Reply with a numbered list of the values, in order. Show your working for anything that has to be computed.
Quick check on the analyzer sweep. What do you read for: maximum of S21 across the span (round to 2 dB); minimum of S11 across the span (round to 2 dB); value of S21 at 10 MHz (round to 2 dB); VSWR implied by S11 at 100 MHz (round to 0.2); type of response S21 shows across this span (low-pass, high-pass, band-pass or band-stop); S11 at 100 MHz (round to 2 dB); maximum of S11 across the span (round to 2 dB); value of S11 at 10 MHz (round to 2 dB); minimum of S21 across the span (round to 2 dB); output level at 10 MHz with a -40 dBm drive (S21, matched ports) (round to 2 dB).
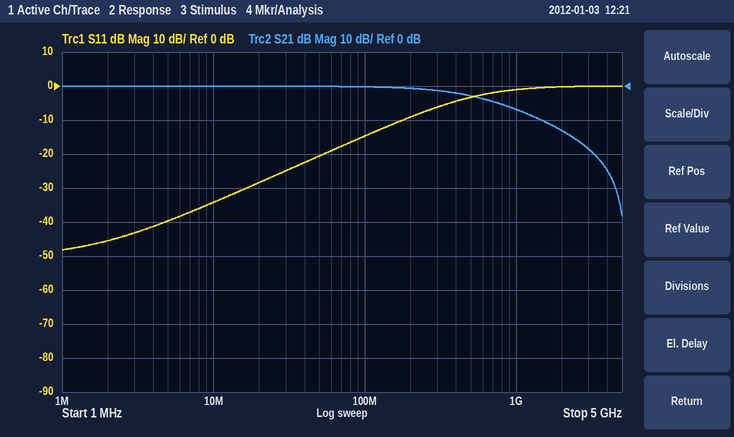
1. 0 dB
2. -48 dB
3. 0 dB
4. |Γ| = 10^(-14/20) = 0.1995; VSWR = (1 + 0.1995)/(1 − 0.1995) ≈ 1.50, so 1.4 to the nearest 0.2
5. low-pass
6. -14 dB
7. 0 dB
8. -34 dB
9. -38 dB
10. -40 dBm + (0 dB) = -40 dBm
